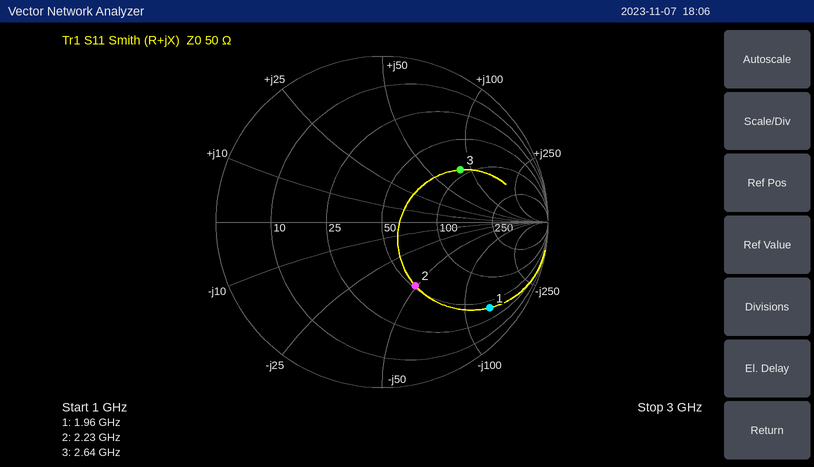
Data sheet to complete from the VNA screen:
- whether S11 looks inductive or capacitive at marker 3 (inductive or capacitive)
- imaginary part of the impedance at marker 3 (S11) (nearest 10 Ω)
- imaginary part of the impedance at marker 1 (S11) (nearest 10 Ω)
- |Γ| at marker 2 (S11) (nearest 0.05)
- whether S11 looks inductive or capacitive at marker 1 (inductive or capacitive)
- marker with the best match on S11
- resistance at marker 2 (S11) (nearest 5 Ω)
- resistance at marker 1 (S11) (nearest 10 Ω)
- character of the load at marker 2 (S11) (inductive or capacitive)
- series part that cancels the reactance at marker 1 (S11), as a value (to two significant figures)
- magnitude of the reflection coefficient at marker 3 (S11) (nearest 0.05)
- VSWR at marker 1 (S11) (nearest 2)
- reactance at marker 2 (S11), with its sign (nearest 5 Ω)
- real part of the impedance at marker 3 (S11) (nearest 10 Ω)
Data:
inductive
+80 Ω
-130 Ω
0.45
capacitive
marker 2
50 Ω
40 Ω
capacitive
11 nH
0.55
10
-50 Ω
90 Ω
